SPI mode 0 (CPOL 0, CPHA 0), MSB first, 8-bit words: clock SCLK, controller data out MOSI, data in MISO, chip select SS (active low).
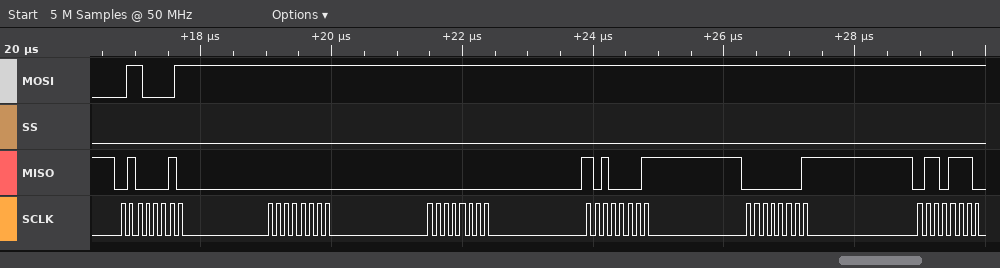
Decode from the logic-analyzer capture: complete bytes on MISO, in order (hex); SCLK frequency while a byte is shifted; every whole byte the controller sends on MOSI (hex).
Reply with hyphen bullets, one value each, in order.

- 42 00 00 A1 01 6E
- 8 MHz
- 61 FF FF FF FF FF
